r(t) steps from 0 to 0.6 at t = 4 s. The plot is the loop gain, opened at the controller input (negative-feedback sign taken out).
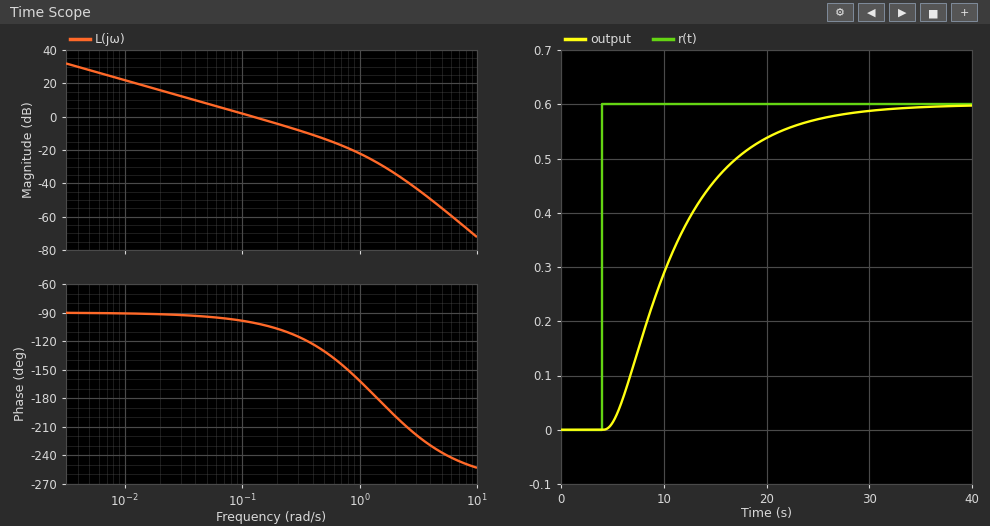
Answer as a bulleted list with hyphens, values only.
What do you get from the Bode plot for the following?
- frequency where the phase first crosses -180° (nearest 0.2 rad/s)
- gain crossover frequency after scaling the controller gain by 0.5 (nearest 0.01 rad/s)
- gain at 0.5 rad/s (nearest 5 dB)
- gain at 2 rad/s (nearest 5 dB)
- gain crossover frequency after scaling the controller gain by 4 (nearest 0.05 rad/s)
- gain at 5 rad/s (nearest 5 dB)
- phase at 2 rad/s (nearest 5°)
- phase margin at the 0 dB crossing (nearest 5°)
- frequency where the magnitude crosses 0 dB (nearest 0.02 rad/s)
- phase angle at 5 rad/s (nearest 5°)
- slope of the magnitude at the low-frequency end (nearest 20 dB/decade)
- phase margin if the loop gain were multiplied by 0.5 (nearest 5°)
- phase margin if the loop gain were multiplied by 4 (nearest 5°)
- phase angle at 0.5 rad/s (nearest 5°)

- 1.4 rad/s
- 0.06 rad/s
- -15 dB
- -35 dB
- 0.45 rad/s
- -55 dB
- -200°
- 80°
- 0.12 rad/s
- -235°
- -20 dB/decade
- 85°
- 55°
- -130°
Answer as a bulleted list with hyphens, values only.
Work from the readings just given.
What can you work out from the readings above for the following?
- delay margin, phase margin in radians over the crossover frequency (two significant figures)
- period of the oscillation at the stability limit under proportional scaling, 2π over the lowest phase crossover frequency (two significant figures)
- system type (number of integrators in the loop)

- 12 s
- 4.5 s
- 1
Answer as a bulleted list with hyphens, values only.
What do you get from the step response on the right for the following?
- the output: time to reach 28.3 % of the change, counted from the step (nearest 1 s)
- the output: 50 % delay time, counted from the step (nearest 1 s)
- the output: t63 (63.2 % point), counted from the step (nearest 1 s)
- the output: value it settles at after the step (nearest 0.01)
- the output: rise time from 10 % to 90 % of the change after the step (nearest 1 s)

- 4 s
- 6 s
- 8 s
- 0.60
- 14 s
